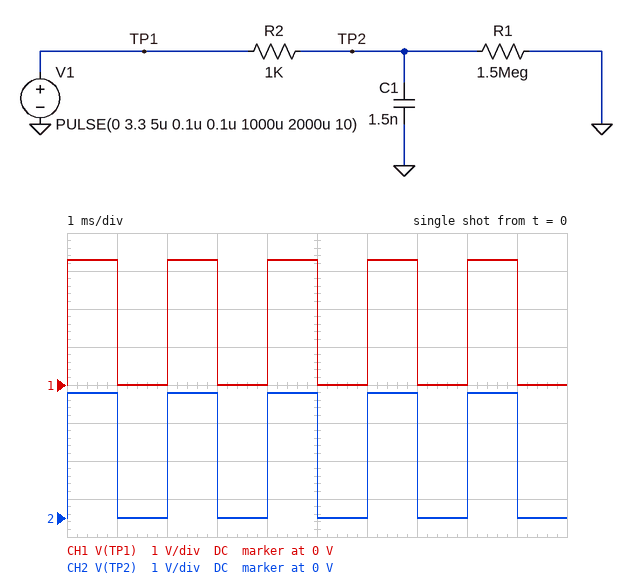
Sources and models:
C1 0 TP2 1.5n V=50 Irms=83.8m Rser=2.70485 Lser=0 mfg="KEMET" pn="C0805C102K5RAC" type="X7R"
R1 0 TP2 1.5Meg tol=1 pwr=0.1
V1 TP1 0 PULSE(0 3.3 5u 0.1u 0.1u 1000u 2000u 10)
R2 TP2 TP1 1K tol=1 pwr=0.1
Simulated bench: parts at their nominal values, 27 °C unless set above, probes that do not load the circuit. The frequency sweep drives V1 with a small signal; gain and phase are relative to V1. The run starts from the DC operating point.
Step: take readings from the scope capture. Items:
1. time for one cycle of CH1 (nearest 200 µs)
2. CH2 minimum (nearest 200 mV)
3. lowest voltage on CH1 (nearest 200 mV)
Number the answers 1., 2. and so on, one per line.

1. 2.0 ms
2. 0 V
3. 0 V
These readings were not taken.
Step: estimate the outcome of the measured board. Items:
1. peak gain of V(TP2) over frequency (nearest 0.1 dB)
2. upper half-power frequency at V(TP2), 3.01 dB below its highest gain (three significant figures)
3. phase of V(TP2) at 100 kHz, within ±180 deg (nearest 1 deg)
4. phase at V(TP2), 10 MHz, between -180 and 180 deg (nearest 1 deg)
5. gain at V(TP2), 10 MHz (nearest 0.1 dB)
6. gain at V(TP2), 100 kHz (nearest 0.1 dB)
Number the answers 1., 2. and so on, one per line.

1. 0 dB
2. 106 kHz
3. -43 deg
4. -75 deg
5. -39.2 dB
6. -2.8 dB
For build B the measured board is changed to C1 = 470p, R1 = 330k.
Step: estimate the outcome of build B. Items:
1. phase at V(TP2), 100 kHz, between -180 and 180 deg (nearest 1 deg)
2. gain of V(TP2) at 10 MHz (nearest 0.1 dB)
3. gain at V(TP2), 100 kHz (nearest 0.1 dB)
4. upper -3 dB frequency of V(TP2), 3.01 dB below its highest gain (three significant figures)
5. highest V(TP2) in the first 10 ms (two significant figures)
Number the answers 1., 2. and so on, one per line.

1. -16 deg
2. -29.4 dB
3. -0.4 dB
4. 339 kHz
5. 3.3 V
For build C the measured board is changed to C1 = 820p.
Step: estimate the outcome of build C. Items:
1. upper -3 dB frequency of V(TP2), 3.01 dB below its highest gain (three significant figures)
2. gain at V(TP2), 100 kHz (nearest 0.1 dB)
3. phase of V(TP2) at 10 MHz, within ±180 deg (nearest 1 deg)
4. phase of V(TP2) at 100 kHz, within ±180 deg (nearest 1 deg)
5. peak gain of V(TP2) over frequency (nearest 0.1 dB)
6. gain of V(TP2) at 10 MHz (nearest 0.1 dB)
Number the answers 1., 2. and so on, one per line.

1. 194 kHz
2. -1.0 dB
3. -81 deg
4. -27 deg
5. 0 dB
6. -34.2 dB
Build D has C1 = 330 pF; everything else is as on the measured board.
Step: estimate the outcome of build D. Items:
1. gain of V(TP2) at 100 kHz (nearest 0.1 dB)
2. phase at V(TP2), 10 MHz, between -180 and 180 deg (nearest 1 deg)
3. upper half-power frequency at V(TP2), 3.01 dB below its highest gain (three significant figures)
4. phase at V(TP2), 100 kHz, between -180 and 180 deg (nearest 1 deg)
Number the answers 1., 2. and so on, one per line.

1. -0.2 dB
2. -84 deg
3. 481 kHz
4. -12 deg
